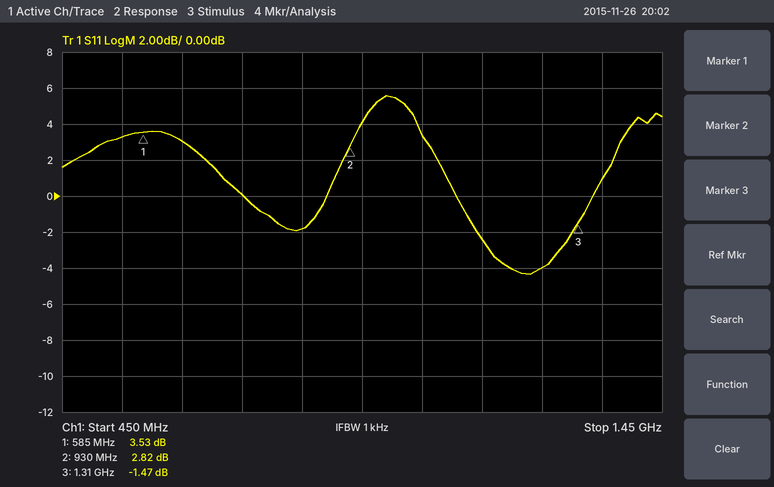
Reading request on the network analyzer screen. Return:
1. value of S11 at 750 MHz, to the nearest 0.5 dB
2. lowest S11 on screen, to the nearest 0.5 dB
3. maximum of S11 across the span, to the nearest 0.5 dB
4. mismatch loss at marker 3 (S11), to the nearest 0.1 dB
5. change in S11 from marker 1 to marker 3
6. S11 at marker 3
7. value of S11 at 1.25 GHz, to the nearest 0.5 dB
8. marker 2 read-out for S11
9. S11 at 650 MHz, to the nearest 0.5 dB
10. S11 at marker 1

0.0 dB
-4.5 dB
5.5 dB
5.4 dB
-5.00 dB
-1.47 dB
-4.0 dB
2.82 dB
3.0 dB
3.53 dB
